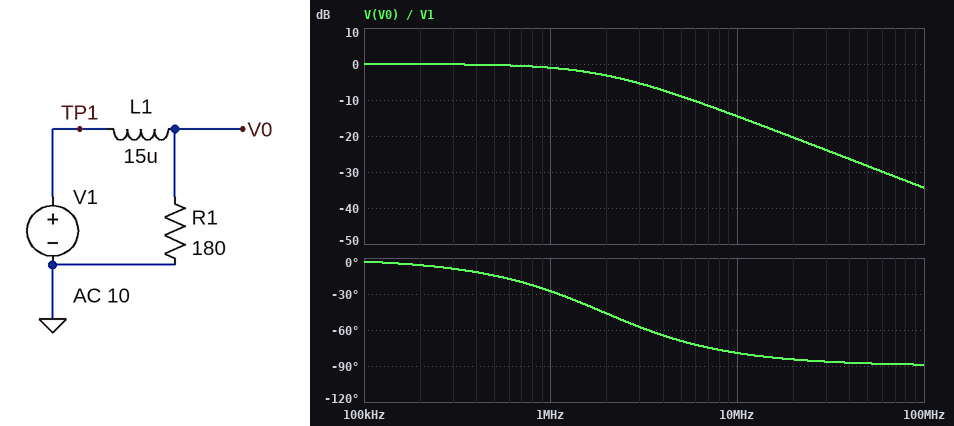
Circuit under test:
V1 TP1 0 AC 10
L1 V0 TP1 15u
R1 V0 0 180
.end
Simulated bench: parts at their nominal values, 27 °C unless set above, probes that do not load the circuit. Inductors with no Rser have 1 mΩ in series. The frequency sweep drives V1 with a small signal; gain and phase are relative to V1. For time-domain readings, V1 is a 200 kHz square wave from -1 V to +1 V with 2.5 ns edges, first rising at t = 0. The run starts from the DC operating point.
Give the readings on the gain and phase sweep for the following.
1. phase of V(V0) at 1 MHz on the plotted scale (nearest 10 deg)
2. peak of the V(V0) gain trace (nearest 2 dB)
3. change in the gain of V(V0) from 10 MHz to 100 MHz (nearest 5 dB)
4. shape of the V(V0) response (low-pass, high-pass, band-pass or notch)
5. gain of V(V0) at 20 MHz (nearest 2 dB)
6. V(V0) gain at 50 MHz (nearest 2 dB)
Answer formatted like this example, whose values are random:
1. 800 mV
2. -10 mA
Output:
1. -30 deg
2. 0 dB
3. -20 dB
4. low-pass
5. -20 dB
6. -28 dB
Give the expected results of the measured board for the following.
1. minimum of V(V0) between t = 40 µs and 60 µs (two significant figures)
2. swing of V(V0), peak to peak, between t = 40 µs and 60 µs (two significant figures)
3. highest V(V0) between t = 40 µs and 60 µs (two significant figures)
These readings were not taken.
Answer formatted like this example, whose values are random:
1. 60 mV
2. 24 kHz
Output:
1. -1.0 V
2. 2.0 V
3. 1.0 V
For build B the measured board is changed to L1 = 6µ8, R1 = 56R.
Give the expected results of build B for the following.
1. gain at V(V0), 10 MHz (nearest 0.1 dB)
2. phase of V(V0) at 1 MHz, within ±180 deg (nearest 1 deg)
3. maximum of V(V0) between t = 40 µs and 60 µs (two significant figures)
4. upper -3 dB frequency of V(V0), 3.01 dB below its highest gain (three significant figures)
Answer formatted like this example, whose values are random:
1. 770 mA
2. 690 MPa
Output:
1. -17.7 dB
2. -37 deg
3. 1.0 V
4. 1.31 MHz
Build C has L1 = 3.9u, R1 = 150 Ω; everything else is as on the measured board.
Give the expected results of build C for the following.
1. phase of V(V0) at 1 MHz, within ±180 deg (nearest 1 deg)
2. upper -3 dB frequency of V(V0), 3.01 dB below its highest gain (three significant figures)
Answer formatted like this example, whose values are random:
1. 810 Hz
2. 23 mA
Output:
1. -9 deg
2. 6.12 MHz
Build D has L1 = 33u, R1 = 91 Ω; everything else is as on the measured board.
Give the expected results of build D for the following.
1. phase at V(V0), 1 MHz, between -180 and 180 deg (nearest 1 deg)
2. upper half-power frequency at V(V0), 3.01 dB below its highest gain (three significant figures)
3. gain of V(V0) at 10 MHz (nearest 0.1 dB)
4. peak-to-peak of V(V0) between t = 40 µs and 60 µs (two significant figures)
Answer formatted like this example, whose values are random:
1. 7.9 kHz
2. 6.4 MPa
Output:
1. -66 deg
2. 439 kHz
3. -27.2 dB
4. 2.0 V
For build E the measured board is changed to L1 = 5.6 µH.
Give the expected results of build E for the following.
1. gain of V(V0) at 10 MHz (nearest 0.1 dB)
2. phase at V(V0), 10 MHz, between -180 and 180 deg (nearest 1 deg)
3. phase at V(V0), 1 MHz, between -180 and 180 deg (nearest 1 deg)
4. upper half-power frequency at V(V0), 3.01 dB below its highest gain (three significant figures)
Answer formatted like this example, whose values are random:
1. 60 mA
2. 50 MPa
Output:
1. -6.8 dB
2. -63 deg
3. -11 deg
4. 5.12 MHz
